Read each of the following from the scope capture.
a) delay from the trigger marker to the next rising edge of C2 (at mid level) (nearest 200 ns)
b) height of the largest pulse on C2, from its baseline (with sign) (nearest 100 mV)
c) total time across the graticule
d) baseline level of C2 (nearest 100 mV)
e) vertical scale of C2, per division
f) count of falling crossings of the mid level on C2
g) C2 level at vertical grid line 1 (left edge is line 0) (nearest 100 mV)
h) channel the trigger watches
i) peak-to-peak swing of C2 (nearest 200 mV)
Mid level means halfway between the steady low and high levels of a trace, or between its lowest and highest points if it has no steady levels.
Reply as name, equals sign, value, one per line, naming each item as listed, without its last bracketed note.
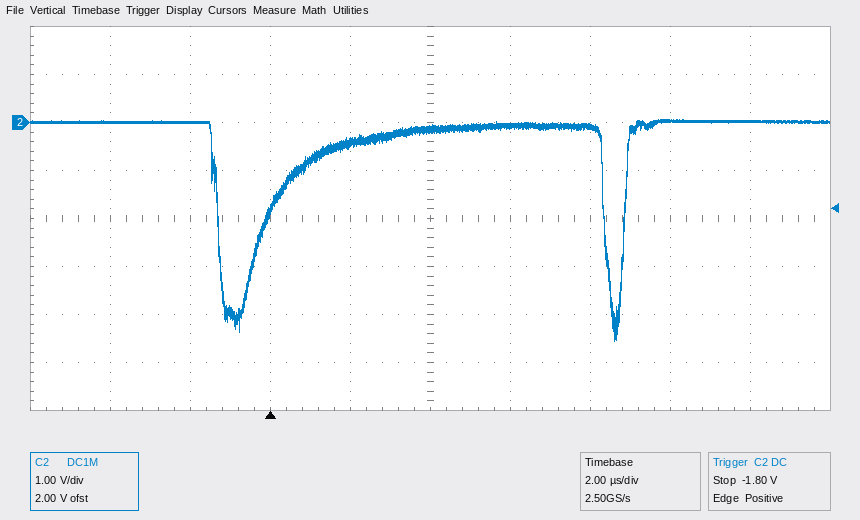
delay from the trigger marker to the next rising edge of C2 (at mid level) = 8.8 µs
height of the largest pulse on C2, from its baseline (with sign) = -4.6 V
total time across the graticule = 20 µs
baseline level of C2 = 0.0 V
vertical scale of C2, per division = 1 V
count of falling crossings of the mid level on C2 = 2
C2 level at vertical grid line 1 (left edge is line 0) = 0.0 V
channel the trigger watches = C2
peak-to-peak swing of C2 = 4.6 V
